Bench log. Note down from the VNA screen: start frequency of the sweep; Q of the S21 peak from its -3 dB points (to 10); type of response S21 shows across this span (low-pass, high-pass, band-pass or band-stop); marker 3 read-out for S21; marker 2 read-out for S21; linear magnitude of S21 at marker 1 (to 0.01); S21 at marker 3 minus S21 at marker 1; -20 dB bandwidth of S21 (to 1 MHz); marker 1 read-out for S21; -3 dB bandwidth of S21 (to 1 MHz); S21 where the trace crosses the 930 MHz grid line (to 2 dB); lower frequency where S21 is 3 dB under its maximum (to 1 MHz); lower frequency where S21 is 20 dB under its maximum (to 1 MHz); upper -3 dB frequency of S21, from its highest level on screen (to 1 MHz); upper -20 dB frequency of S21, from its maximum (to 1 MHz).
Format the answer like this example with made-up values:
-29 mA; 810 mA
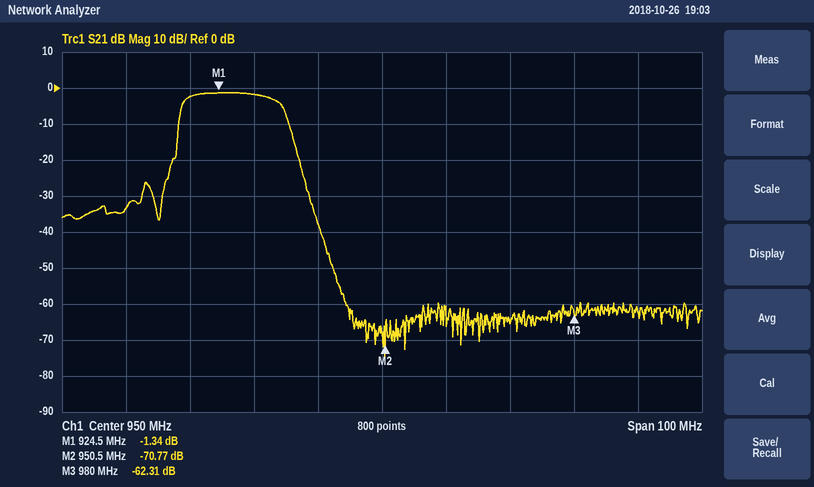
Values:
900 MHz; 60; band-pass; -62.31 dB; -70.77 dB; 0.86; -60.97 dB; 20 MHz; -1.34 dB; 15 MHz; -2 dB; 919 MHz; 917 MHz; 934 MHz; 937 MHz
